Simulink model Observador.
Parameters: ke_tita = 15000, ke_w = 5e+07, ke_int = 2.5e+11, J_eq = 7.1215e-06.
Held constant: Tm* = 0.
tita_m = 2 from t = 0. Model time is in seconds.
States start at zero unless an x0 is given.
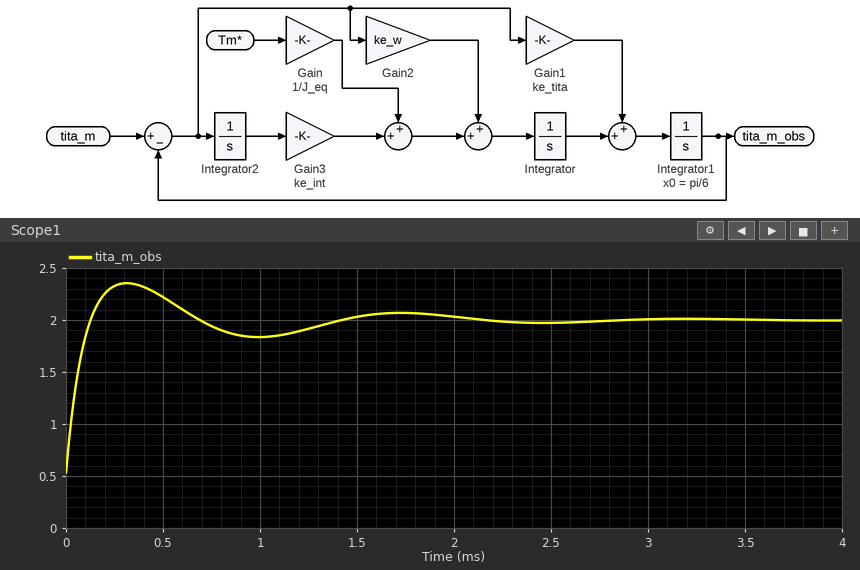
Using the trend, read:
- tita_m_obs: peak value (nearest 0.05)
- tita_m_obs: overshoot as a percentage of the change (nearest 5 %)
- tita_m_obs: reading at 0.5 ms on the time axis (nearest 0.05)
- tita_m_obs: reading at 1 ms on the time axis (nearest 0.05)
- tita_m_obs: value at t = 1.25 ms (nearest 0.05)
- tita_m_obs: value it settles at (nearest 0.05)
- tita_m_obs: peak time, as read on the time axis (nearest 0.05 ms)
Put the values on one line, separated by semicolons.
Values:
2.35; 25 %; 2.20; 1.85; 1.90; 2.00; 0.30 ms
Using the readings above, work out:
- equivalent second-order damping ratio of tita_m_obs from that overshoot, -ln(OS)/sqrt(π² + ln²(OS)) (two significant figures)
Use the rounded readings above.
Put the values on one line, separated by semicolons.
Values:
0.40
